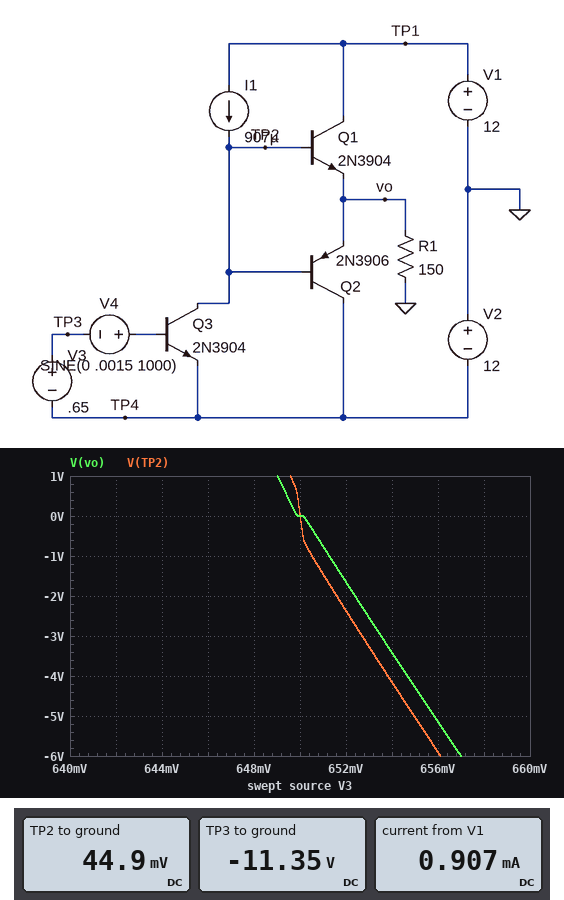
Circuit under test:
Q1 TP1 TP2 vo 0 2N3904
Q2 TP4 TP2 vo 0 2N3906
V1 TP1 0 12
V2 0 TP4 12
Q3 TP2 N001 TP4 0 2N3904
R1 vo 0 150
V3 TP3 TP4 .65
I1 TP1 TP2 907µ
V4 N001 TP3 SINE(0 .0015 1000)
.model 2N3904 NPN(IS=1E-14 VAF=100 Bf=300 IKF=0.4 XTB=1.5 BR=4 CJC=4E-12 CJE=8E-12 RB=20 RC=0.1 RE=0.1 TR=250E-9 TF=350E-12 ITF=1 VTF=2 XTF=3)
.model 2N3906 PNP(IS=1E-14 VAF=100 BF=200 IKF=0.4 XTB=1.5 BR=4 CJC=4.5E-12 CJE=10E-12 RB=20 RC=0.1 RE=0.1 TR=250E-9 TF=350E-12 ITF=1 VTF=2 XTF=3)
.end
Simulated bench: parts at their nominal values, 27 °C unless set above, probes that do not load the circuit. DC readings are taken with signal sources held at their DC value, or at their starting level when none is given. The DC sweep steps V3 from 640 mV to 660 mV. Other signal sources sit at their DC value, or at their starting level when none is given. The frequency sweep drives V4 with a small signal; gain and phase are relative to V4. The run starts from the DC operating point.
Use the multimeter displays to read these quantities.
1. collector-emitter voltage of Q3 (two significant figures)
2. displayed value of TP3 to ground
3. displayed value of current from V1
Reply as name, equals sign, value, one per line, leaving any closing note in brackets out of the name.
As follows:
collector-emitter voltage of Q3 = 12 V
displayed value of TP3 to ground = -11.35 V
displayed value of current from V1 = 0.907 mA
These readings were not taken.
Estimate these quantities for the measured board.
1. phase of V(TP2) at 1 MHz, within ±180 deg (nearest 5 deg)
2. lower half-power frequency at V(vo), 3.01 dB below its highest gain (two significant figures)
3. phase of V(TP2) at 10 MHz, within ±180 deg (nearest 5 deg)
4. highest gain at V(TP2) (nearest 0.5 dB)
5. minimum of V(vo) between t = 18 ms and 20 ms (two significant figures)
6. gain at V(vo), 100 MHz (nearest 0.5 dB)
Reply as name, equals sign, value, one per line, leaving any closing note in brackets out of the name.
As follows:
phase of V(TP2) at 1 MHz, within ±180 deg = 95 deg
lower half-power frequency at V(vo), 3.01 dB below its highest gain = 54 kHz
phase of V(TP2) at 10 MHz, within ±180 deg = 95 deg
highest gain at V(TP2) = 72.5 dB
minimum of V(vo) between t = 18 ms and 20 ms = -1.2 V
gain at V(vo), 100 MHz = 10.5 dB
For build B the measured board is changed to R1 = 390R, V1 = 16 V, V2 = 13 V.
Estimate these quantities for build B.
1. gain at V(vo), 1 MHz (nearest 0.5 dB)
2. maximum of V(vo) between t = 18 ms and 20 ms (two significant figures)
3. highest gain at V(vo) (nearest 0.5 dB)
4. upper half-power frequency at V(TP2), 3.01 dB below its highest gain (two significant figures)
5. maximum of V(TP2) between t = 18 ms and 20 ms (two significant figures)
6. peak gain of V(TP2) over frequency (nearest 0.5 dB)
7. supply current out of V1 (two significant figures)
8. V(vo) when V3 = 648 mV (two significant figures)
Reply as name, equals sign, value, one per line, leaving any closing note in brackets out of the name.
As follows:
gain at V(vo), 1 MHz = 53.0 dB
maximum of V(vo) between t = 18 ms and 20 ms = 2.5 V
highest gain at V(vo) = 64.5 dB
upper half-power frequency at V(TP2), 3.01 dB below its highest gain = 280 kHz
maximum of V(TP2) between t = 18 ms and 20 ms = 3.2 V
peak gain of V(TP2) over frequency = 66.0 dB
supply current out of V1 = 910 µA
V(vo) when V3 = 648 mV = 3.6 V
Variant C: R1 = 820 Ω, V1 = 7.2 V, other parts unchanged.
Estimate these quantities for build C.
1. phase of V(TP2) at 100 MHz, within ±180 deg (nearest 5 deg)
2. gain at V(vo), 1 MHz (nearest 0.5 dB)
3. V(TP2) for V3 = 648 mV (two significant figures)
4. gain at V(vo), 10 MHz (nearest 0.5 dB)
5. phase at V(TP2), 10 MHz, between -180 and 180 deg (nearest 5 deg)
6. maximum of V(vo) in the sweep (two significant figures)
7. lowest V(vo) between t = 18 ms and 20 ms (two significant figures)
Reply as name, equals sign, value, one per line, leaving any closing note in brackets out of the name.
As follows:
phase of V(TP2) at 100 MHz, within ±180 deg = 90 deg
gain at V(vo), 1 MHz = 26.5 dB
V(TP2) for V3 = 648 mV = 6.1 V
gain at V(vo), 10 MHz = 26.0 dB
phase at V(TP2), 10 MHz, between -180 and 180 deg = 120 deg
maximum of V(vo) in the sweep = 7.1 V
lowest V(vo) between t = 18 ms and 20 ms = -3.3 V
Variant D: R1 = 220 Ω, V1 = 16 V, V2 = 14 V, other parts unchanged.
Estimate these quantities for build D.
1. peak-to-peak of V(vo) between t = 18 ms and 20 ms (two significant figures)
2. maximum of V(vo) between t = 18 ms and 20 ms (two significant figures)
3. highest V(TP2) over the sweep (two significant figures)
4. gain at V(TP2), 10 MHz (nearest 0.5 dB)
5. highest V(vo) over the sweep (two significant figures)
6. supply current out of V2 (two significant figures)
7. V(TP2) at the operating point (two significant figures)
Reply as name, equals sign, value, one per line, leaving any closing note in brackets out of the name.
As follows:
peak-to-peak of V(vo) between t = 18 ms and 20 ms = 3.6 V
maximum of V(vo) between t = 18 ms and 20 ms = 1.4 V
highest V(TP2) over the sweep = 13 V
gain at V(TP2), 10 MHz = 36.0 dB
highest V(vo) over the sweep = 12 V
supply current out of V2 = 2.6 mA
V(TP2) at the operating point = -1.0 V
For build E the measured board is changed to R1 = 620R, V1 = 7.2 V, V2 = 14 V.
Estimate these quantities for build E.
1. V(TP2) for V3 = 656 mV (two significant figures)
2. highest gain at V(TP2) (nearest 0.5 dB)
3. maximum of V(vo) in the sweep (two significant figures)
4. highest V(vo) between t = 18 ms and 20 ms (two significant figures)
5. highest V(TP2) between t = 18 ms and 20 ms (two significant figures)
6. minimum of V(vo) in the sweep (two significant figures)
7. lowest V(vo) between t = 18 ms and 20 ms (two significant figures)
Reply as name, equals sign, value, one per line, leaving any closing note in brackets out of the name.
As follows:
V(TP2) for V3 = 656 mV = -14 V
highest gain at V(TP2) = 67.5 dB
maximum of V(vo) in the sweep = 7.1 V
highest V(vo) between t = 18 ms and 20 ms = 2.4 V
highest V(TP2) between t = 18 ms and 20 ms = 3.1 V
minimum of V(vo) in the sweep = -13 V
lowest V(vo) between t = 18 ms and 20 ms = -4.0 V
